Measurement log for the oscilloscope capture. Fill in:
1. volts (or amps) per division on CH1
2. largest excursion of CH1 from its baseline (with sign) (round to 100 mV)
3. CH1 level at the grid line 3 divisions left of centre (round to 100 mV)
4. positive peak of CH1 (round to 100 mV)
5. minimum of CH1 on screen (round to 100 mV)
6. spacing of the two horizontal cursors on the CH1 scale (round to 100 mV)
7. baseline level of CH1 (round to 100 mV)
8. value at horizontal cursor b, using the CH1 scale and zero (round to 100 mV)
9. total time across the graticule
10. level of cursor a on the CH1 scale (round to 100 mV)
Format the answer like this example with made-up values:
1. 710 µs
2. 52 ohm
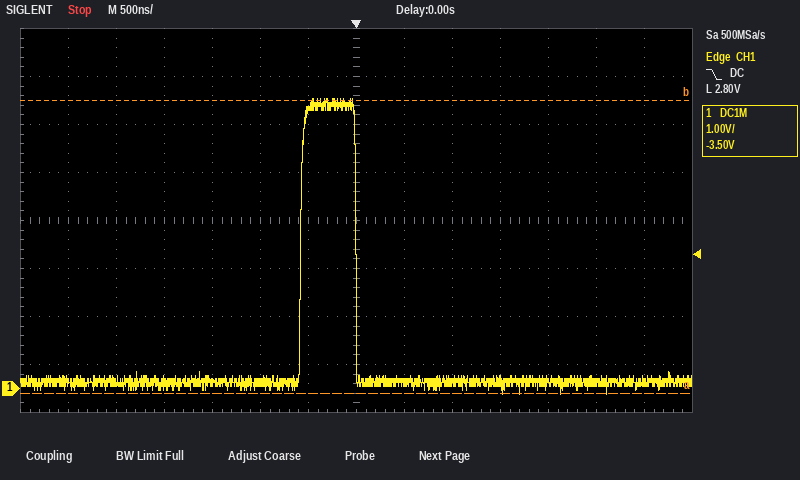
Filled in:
1. 1 V
2. +5.9 V
3. 100 mV
4. 6.0 V
5. -100 mV
6. 6.1 V
7. 100 mV
8. 6.0 V
9. 7 µs
10. -100 mV
